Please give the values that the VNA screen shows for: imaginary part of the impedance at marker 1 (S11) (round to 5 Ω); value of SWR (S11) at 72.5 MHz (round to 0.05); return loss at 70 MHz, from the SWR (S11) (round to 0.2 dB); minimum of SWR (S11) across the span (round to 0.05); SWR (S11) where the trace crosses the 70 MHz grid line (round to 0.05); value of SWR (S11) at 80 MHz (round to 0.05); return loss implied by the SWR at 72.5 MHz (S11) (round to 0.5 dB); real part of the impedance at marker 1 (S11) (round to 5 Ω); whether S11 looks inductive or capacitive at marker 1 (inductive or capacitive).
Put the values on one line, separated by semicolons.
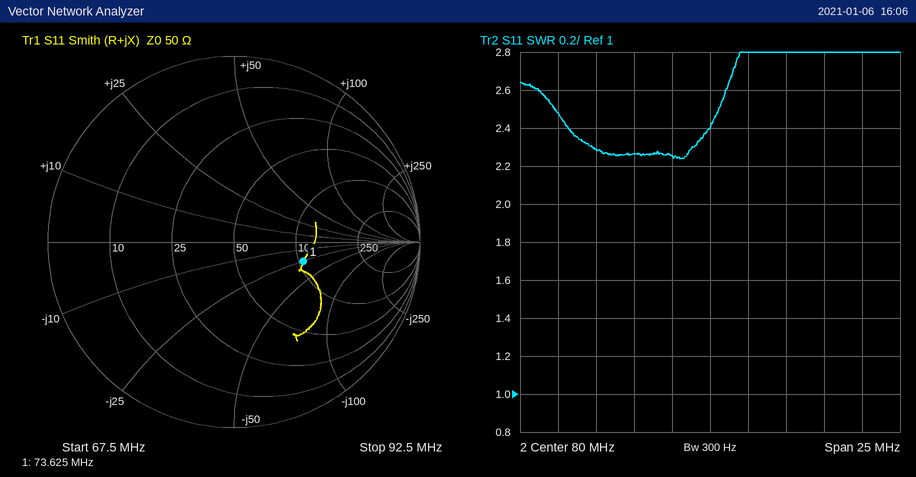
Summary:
-25 Ω; 2.30; 7.4 dB; 2.25; 2.50; 2.40; 8.0 dB; 105 Ω; capacitive
